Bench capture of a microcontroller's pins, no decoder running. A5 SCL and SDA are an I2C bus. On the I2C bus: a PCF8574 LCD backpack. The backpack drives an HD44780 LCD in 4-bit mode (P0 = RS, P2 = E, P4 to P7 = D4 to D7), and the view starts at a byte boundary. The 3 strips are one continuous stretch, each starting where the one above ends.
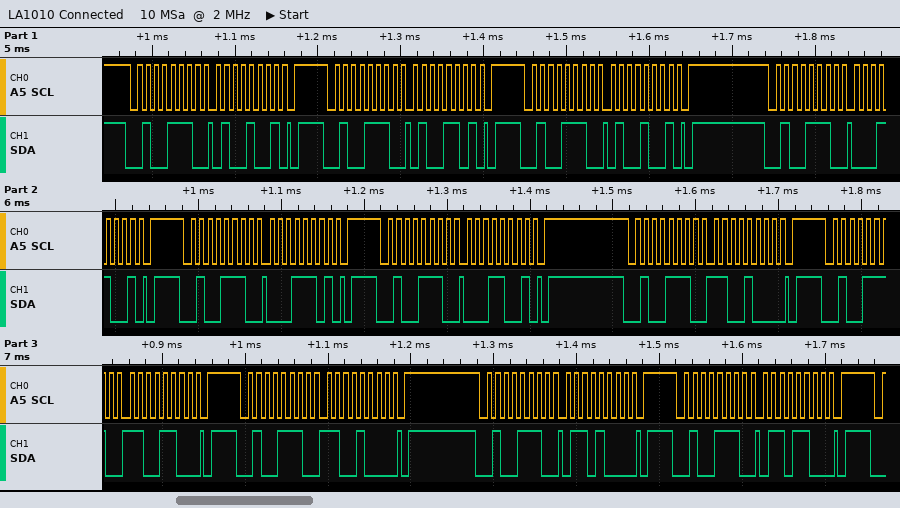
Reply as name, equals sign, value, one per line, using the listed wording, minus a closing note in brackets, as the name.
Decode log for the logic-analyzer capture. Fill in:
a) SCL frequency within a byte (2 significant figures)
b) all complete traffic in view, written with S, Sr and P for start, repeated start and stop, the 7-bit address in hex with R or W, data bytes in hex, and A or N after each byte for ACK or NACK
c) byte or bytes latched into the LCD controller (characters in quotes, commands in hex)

SCL frequency within a byte = 100 kHz
all complete traffic in view, written with S, Sr and P for start, repeated start and stop, the 7-bit address in hex with R or W, data bytes in hex, and A or N after each byte for ACK or NACK = S 27W A 49 A P S 27W A 4D A P S 27W A 49 A P S 27W A 19 A P S 27W A 1D A P S 27W A 19 A P S 27W A C8 A P S 27W A CC A P S 27W A C8 A P S 27W A 68 A P S 27W A 6C A P
byte or bytes latched into the LCD controller = 'A'
